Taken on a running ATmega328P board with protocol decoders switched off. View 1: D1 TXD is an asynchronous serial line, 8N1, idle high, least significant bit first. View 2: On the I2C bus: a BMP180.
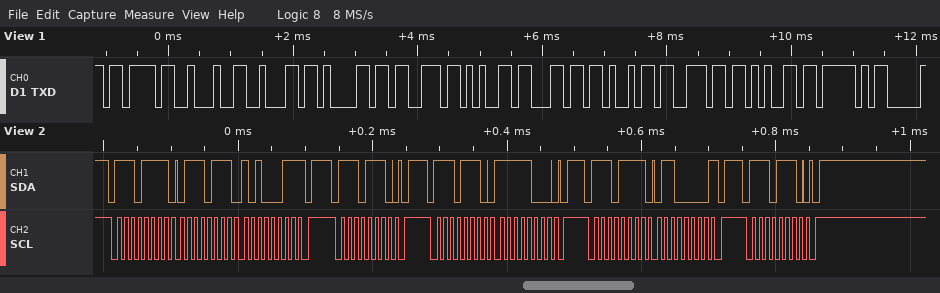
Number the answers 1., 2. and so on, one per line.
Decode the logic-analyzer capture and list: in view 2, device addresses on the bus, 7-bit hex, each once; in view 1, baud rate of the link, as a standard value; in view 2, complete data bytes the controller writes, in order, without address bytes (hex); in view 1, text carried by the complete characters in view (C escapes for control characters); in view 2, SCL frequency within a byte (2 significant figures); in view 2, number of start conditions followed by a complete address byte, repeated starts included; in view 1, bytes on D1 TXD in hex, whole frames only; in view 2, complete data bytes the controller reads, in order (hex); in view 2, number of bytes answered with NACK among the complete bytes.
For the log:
1. 0x77
2. 9600 baud
3. F8
4. "{\"baseline_"
5. 100 kHz
6. 5
7. 0x7B 0x22 0x62 0x61 0x73 0x65 0x6C 0x69 0x6E 0x65 0x5F
8. 77 A3 60
9. 2
